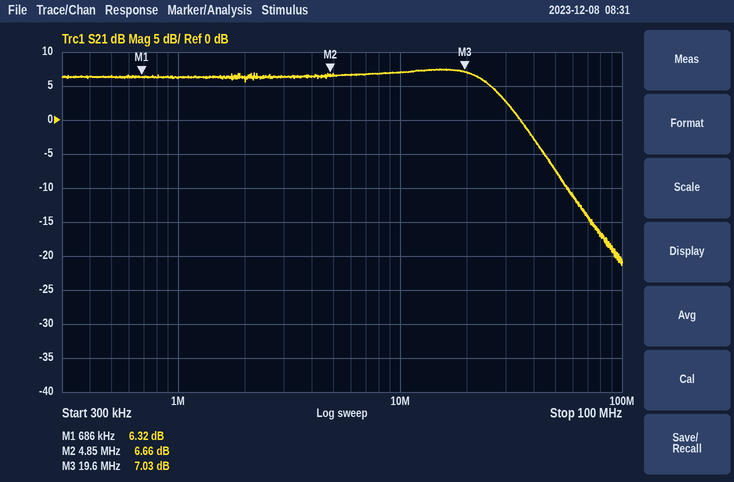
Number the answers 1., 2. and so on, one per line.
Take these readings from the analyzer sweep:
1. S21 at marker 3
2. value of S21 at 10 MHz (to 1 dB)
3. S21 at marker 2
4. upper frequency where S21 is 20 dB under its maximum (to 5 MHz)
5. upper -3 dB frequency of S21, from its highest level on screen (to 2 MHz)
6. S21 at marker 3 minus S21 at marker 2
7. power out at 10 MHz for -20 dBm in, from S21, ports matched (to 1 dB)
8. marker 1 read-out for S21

1. 7.03 dB
2. 7 dB
3. 6.66 dB
4. 65 MHz
5. 26 MHz
6. 0.37 dB
7. -13 dBm
8. 6.32 dB
